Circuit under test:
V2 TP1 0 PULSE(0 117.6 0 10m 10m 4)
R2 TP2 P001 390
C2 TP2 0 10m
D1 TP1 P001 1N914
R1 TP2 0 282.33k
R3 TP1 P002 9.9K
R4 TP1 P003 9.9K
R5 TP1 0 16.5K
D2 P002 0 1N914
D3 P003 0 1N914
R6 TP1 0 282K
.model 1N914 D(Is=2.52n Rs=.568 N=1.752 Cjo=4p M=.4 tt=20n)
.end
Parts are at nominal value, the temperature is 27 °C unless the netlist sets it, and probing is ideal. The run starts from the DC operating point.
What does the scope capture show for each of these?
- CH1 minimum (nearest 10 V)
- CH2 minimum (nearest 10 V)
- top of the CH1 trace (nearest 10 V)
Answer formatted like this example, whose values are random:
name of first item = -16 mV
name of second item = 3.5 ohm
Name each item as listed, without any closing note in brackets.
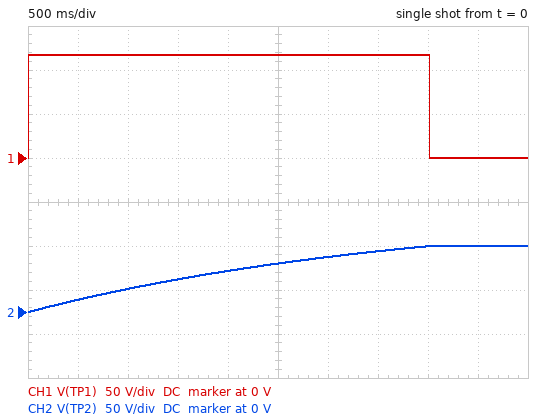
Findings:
CH1 minimum = 0 V
CH2 minimum = 0 V
top of the CH1 trace = 120 V
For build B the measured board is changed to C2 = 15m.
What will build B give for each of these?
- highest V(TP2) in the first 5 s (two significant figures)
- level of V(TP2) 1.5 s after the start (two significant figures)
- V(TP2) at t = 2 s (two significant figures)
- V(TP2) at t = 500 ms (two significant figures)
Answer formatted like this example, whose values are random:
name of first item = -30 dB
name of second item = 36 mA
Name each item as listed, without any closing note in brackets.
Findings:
highest V(TP2) in the first 5 s = 58 V
level of V(TP2) 1.5 s after the start = 26 V
V(TP2) at t = 2 s = 34 V
V(TP2) at t = 500 ms = 9.5 V
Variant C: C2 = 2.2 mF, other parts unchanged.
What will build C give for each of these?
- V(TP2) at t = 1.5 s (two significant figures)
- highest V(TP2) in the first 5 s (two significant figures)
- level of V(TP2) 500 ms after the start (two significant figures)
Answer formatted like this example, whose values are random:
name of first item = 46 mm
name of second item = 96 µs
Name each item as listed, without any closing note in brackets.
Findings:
V(TP2) at t = 1.5 s = 96 V
highest V(TP2) in the first 5 s = 120 V
level of V(TP2) 500 ms after the start = 51 V
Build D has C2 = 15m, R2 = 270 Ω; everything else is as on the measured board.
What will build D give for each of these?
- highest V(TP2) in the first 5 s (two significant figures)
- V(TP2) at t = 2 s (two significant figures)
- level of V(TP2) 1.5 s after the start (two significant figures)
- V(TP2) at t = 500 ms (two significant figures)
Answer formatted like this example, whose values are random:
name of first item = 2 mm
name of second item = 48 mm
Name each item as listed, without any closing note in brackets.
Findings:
highest V(TP2) in the first 5 s = 73 V
V(TP2) at t = 2 s = 45 V
level of V(TP2) 1.5 s after the start = 36 V
V(TP2) at t = 500 ms = 13 V
